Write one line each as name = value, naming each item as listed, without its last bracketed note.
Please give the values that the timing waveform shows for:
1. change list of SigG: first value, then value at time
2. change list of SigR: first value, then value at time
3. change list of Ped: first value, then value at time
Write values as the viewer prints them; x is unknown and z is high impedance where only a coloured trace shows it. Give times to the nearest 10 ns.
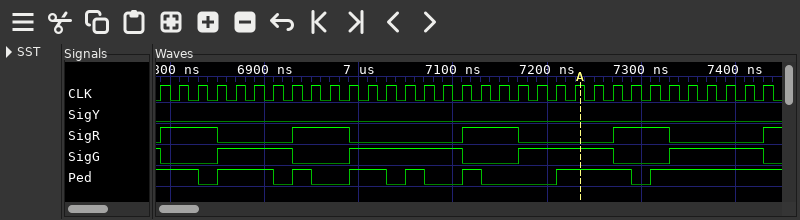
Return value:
change list of SigG: first value, then value at time = 1, 0 at 6790 ns, 1 at 6850 ns, 0 at 6930 ns, 1 at 6990 ns, 0 at 7110 ns, 1 at 7170 ns, 0 at 7270 ns, 1 at 7330 ns, 0 at 7430 ns
change list of SigR: first value, then value at time = 0, 1 at 6790 ns, 0 at 6850 ns, 1 at 6930 ns, 0 at 6990 ns, 1 at 7110 ns, 0 at 7170 ns, 1 at 7270 ns, 0 at 7330 ns, 1 at 7430 ns
change list of Ped: first value, then value at time = 1, 0 at 6830 ns, 1 at 6850 ns, 0 at 6910 ns, 1 at 6930 ns, 0 at 6950 ns, 1 at 6990 ns, 0 at 7030 ns, 1 at 7050 ns, 0 at 7070 ns, 1 at 7110 ns, 0 at 7130 ns, 1 at 7210 ns, 0 at 7290 ns, 1 at 7310 ns
